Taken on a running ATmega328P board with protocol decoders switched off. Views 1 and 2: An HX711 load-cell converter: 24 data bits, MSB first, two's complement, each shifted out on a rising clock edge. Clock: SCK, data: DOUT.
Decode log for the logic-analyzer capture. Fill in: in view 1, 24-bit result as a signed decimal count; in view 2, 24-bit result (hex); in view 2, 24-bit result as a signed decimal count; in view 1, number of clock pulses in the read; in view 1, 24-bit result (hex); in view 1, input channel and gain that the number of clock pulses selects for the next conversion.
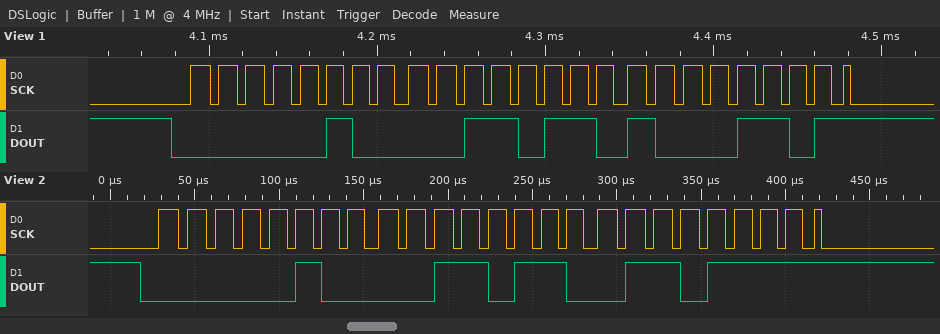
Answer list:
276109
0x04366F
276079
25
0x04368D
channel A, gain 128
